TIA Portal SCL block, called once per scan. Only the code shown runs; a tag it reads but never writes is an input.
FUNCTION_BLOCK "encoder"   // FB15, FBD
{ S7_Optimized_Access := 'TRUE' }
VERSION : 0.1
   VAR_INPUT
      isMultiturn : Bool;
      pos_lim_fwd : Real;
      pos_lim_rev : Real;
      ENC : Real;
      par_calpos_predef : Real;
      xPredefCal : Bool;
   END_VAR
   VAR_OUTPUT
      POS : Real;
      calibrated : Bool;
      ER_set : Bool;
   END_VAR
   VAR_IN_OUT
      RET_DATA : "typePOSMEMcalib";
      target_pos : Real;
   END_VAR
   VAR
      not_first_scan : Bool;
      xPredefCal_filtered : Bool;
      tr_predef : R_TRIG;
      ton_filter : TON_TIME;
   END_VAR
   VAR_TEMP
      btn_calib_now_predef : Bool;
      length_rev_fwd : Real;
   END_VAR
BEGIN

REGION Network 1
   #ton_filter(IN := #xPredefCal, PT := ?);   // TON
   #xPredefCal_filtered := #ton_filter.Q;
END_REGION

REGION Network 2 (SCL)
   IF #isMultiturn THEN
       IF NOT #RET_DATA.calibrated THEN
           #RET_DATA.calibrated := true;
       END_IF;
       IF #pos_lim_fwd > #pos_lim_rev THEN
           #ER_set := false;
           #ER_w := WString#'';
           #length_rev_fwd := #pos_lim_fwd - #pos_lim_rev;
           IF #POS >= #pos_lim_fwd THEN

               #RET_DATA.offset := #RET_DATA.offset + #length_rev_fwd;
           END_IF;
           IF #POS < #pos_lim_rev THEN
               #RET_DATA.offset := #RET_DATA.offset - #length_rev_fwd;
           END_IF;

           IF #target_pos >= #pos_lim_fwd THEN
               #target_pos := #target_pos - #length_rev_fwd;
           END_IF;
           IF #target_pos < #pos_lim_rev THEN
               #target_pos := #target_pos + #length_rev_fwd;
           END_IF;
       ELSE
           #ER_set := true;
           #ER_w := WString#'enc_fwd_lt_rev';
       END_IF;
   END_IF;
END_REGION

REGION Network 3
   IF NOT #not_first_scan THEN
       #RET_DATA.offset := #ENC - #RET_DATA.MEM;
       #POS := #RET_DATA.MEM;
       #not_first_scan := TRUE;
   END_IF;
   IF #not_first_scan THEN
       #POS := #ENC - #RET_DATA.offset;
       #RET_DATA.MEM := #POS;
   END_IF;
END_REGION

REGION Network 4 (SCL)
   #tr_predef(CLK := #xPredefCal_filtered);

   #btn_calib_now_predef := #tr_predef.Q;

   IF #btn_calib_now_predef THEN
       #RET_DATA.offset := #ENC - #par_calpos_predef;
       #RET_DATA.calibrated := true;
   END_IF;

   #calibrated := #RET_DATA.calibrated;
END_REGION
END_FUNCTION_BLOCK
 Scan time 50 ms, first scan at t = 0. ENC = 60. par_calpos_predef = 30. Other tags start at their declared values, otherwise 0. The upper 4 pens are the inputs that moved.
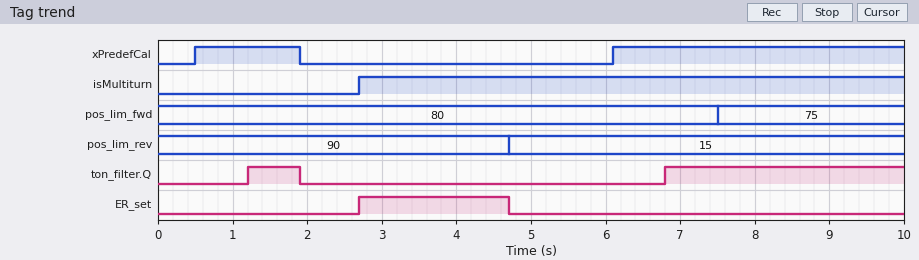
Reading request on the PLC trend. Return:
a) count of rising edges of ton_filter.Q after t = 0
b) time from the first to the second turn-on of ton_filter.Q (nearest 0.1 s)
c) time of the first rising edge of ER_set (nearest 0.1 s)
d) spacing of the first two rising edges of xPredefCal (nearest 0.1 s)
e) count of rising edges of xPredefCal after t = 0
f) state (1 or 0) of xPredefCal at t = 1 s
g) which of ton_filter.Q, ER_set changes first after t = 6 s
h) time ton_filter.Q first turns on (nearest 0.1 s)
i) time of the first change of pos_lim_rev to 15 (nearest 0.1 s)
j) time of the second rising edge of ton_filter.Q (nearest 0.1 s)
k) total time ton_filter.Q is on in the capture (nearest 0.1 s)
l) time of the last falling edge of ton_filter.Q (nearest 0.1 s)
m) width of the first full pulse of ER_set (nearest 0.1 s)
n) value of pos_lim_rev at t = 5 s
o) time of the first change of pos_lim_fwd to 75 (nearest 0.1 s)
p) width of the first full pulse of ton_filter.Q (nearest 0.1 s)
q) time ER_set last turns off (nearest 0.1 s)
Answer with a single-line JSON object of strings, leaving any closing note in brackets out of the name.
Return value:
{"count of rising edges of ton_filter.Q after t = 0": "2", "time from the first to the second turn-on of ton_filter.Q": "5.6 s", "time of the first rising edge of ER_set": "2.7 s", "spacing of the first two rising edges of xPredefCal": "5.6 s", "count of rising edges of xPredefCal after t = 0": "2", "state (1 or 0) of xPredefCal at t = 1 s": "1", "which of ton_filter.Q, ER_set changes first after t = 6 s": "ton_filter.Q", "time ton_filter.Q first turns on": "1.2 s", "time of the first change of pos_lim_rev to 15": "4.7 s", "time of the second rising edge of ton_filter.Q": "6.8 s", "total time ton_filter.Q is on in the capture": "3.9 s", "time of the last falling edge of ton_filter.Q": "1.9 s", "width of the first full pulse of ER_set": "2.0 s", "value of pos_lim_rev at t = 5 s": "15", "time of the first change of pos_lim_fwd to 75": "7.5 s", "width of the first full pulse of ton_filter.Q": "0.7 s", "time ER_set last turns off": "4.7 s"}
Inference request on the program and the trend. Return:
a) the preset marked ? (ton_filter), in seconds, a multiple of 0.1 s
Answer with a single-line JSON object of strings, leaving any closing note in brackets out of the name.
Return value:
{"the preset marked ? (ton_filter), in seconds, a multiple of 0.1 s": "0.7 s"}
